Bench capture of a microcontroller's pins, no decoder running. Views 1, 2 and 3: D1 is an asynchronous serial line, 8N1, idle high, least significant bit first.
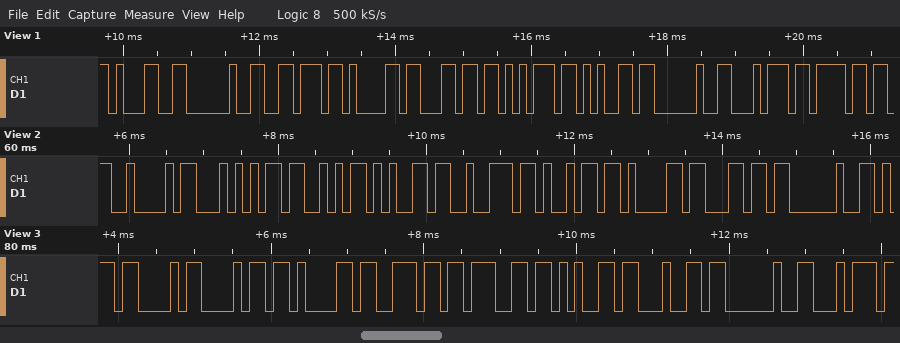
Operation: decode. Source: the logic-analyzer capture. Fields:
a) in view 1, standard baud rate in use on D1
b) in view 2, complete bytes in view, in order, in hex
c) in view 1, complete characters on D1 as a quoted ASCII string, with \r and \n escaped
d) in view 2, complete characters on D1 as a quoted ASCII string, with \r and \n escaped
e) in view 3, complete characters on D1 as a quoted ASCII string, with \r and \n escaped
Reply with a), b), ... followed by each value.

a) 9600 baud
b) 42 54 53 65 72 69 61 6C 20
c) "1 value to"
d) "BTSerial "
e) "Changed t"
